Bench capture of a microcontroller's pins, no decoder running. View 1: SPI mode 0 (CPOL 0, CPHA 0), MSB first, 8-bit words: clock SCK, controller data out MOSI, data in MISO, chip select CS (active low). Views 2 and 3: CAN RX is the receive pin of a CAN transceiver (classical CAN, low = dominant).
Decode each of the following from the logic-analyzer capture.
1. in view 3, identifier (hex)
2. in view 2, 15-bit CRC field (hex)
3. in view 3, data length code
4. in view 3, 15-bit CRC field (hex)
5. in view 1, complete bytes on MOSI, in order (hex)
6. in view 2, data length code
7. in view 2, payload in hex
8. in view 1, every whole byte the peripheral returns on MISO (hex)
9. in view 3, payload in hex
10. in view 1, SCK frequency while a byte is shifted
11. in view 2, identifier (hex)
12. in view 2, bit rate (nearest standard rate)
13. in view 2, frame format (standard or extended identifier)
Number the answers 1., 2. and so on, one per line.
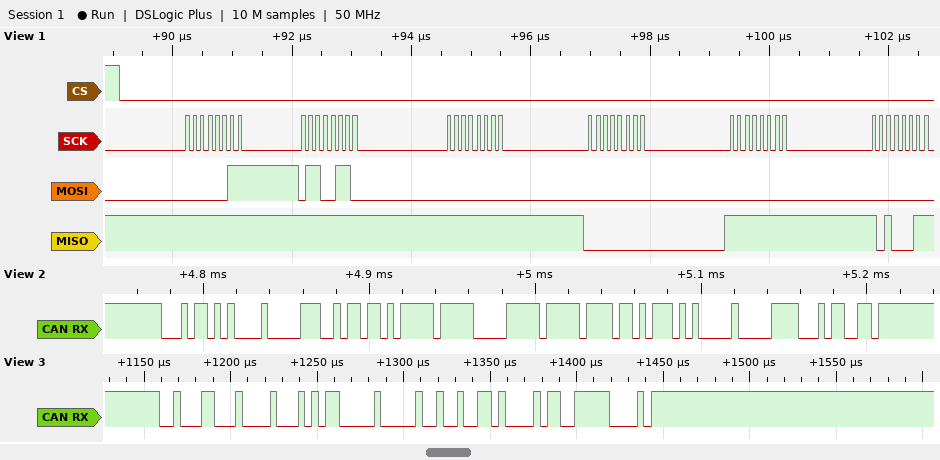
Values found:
1. 0x231
2. 0x1C59
3. 4
4. 0x2CF8
5. 03 66 00 00 00 00
6. 8
7. 32 DA FF C3 FF ED 75 00
8. FF FF FF 00 FF A3
9. 56 00 12 68
10. 8 MHz
11. 0x16A
12. 250 kbit/s
13. standard
